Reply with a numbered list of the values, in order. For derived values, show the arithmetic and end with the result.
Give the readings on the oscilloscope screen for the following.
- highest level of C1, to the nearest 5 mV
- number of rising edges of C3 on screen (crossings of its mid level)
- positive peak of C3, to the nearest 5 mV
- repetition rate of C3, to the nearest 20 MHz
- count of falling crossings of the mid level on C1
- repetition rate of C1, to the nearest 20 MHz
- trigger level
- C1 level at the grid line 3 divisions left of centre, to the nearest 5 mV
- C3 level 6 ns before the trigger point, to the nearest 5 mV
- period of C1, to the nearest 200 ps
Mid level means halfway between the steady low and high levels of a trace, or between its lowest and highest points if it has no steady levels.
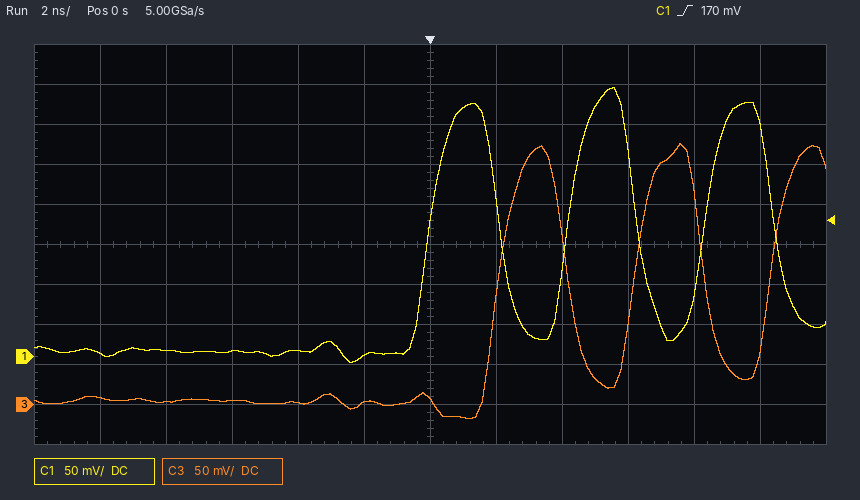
1. 335 mV
2. 3
3. 325 mV
4. 240 MHz
5. 3
6. 1 / 4.2 ns ≈ 238 MHz, so 240 MHz to the nearest 20 MHz
7. 170 mV
8. 5 mV
9. 5 mV
10. 4.2 ns
